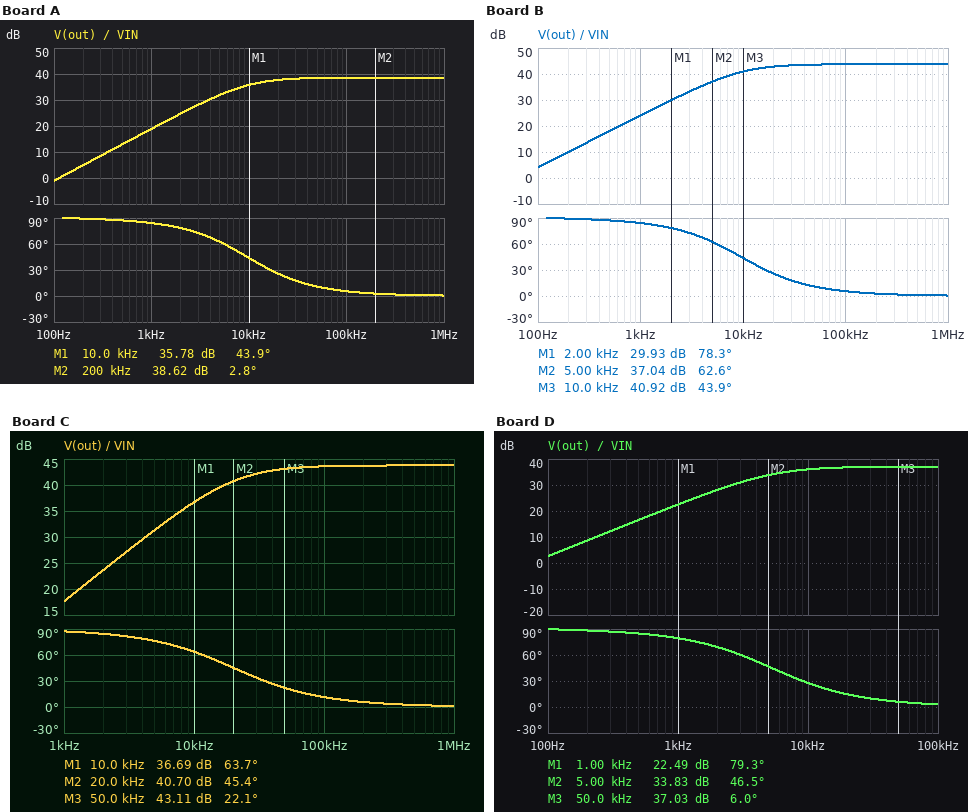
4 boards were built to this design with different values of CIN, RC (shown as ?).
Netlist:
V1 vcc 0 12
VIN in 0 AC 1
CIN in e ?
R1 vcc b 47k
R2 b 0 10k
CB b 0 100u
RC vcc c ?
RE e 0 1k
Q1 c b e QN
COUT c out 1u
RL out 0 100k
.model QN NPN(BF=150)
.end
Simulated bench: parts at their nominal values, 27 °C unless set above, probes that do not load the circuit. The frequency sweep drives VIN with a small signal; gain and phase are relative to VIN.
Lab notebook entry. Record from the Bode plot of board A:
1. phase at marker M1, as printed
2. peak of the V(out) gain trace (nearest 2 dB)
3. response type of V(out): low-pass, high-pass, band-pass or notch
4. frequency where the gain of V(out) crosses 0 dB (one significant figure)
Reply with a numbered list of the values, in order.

1. 43.9 deg
2. 38 dB
3. high-pass
4. 100 Hz
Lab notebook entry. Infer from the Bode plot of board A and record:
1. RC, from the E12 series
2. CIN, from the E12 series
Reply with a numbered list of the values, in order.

1. 1.8 kΩ
2. 820 nF
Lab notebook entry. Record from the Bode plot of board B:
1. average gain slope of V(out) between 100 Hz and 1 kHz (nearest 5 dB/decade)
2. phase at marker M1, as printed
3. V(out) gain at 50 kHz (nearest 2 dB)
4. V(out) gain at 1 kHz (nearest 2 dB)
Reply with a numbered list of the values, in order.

1. 20 dB/decade
2. 78.3 deg
3. 44 dB
4. 24 dB
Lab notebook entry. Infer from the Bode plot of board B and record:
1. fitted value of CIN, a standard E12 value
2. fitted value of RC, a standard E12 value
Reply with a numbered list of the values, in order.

1. 820 nF
2. 3.3 kΩ
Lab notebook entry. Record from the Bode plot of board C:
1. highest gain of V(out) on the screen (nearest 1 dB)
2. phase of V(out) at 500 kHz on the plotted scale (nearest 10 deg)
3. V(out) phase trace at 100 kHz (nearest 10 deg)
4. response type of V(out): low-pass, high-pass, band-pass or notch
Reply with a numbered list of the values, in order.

1. 44 dB
2. 0 deg
3. 10 deg
4. high-pass
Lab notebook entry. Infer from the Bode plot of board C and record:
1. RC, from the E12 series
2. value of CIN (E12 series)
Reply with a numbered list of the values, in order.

1. 3.3 kΩ
2. 390 nF
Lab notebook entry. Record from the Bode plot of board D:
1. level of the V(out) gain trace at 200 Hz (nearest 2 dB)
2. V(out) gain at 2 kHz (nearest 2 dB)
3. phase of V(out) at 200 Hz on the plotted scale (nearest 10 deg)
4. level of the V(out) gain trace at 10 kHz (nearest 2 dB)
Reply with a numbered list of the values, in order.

1. 8 dB
2. 28 dB
3. 90 deg
4. 36 dB
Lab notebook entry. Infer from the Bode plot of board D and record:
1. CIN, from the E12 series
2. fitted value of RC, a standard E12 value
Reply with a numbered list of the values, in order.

1. 1.5 µF
2. 1.5 kΩ
